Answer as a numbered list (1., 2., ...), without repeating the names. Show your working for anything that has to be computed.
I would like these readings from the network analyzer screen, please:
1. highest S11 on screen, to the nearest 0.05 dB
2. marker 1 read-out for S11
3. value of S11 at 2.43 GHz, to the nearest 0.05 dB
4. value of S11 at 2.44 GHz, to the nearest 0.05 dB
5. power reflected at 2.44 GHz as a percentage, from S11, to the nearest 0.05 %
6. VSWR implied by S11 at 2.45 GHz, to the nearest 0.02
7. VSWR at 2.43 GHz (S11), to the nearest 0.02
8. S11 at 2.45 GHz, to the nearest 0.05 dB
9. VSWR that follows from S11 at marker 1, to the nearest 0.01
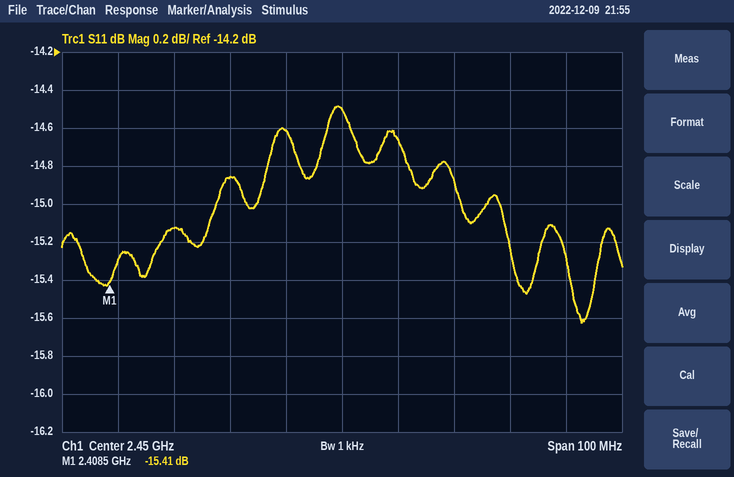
1. -14.50 dB
2. -15.41 dB
3. -14.85 dB
4. -14.60 dB
5. 10^(-14.6/10) ≈ 3.47 %, so 3.45 % to the nearest 0.05 %
6. |Γ| = 10^(-14.5/20) = 0.1884; VSWR = (1 + 0.1884)/(1 − 0.1884) ≈ 1.46
7. |Γ| = 10^(-14.85/20) = 0.1809; VSWR = (1 + 0.1809)/(1 − 0.1809) ≈ 1.44
8. -14.50 dB
9. (1 + 0.1696)/(1 − 0.1696) ≈ 1.41
